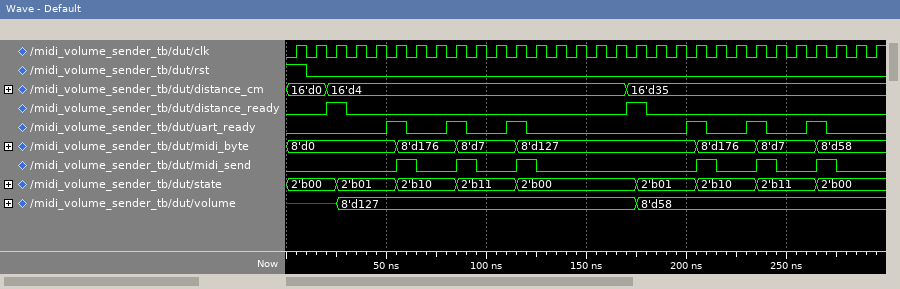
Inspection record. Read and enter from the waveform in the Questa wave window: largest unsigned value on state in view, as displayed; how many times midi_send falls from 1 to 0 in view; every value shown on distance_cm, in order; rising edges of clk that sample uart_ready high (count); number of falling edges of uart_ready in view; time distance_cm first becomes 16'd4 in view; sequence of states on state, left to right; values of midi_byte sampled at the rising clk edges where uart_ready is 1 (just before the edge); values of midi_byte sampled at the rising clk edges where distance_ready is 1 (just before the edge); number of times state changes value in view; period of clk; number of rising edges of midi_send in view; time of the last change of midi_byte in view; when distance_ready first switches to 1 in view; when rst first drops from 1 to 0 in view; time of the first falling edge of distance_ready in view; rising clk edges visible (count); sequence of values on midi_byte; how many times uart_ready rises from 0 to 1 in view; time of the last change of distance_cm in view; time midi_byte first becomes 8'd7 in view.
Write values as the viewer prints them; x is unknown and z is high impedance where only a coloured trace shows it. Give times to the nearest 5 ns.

2'b11
6
16'd0, 16'd4, 16'd35
6
6
20 ns
2'b00, 2'b01, 2'b10, 2'b11, 2'b00, 2'b01, 2'b10, 2'b11, 2'b00
8'd0, 8'd176, 8'd7, 8'd127, 8'd176, 8'd7
8'd0, 8'd127
8
10 ns
6
265 ns
20 ns
10 ns
30 ns
30
8'd0, 8'd176, 8'd7, 8'd127, 8'd176, 8'd7, 8'd58
6
170 ns
85 ns
